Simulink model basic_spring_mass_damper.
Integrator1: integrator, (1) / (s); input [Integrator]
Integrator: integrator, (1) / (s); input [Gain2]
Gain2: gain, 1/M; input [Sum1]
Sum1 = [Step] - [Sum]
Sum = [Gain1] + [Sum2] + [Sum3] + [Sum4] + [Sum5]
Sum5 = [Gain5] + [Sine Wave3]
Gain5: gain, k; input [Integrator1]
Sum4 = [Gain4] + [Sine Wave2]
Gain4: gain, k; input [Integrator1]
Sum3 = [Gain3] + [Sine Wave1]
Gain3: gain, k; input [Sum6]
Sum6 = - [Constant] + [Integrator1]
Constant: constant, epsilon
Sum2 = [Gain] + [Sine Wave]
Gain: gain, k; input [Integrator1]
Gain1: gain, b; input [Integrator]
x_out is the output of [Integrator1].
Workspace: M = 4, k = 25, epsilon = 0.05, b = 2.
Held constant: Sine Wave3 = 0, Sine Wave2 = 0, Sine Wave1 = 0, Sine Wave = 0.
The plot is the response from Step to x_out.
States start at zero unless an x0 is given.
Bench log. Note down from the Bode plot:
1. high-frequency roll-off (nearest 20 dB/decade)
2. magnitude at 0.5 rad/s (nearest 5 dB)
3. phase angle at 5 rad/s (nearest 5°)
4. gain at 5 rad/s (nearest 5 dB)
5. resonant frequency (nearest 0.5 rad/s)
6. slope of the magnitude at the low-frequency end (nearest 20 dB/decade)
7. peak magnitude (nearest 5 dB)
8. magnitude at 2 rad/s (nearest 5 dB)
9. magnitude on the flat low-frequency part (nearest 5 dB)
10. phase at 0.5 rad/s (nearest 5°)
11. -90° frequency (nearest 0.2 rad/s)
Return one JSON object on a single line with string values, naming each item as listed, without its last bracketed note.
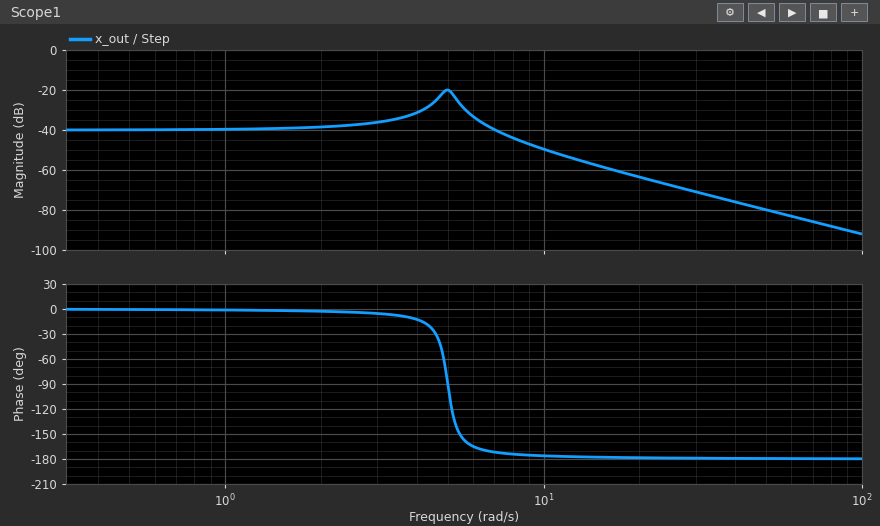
{"high-frequency roll-off": "-40 dB/decade", "magnitude at 0.5 rad/s": "-40 dB", "phase angle at 5 rad/s": "-90°", "gain at 5 rad/s": "-20 dB", "resonant frequency": "5.0 rad/s", "slope of the magnitude at the low-frequency end": "0 dB/decade", "peak magnitude": "-20 dB", "magnitude at 2 rad/s": "-40 dB", "magnitude on the flat low-frequency part": "-40 dB", "phase at 0.5 rad/s": "0°", "-90° frequency": "5.0 rad/s"}
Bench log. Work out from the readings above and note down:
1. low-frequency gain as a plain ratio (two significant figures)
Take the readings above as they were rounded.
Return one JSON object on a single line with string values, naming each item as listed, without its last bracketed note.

{"low-frequency gain as a plain ratio": "0.010"}
